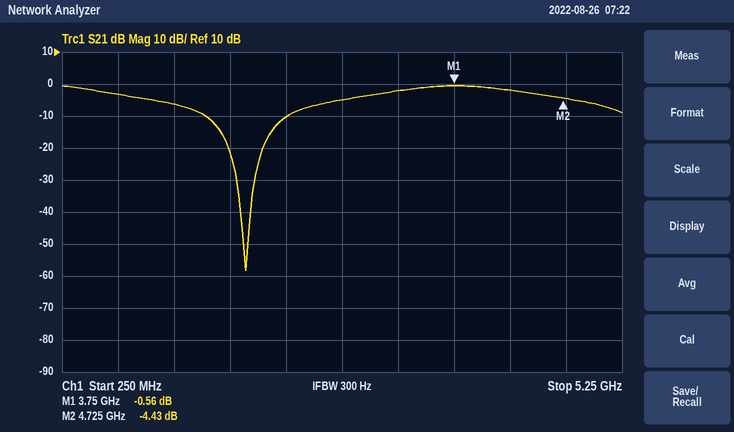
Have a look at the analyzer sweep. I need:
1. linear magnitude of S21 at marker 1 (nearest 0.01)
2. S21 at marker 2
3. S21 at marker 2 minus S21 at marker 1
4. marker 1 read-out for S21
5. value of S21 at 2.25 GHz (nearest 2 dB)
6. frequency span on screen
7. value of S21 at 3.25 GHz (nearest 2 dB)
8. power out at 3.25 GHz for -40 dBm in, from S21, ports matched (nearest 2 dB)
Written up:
0.94
-4.43 dB
-3.87 dB
-0.56 dB
-10 dB
5 GHz
-2 dB
-42 dBm
